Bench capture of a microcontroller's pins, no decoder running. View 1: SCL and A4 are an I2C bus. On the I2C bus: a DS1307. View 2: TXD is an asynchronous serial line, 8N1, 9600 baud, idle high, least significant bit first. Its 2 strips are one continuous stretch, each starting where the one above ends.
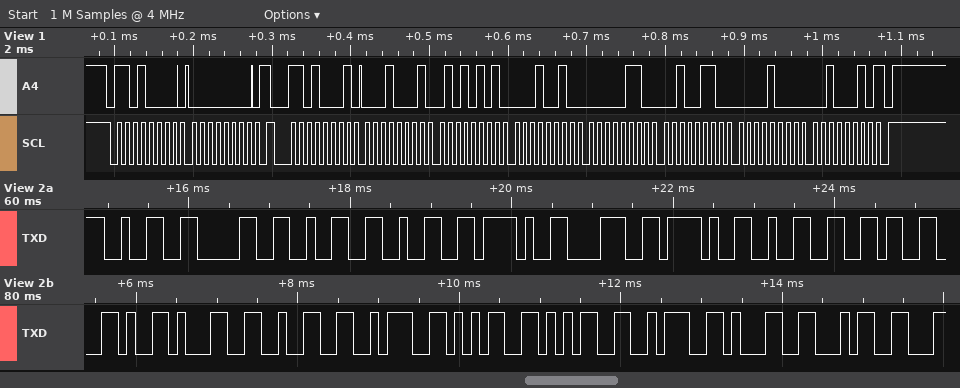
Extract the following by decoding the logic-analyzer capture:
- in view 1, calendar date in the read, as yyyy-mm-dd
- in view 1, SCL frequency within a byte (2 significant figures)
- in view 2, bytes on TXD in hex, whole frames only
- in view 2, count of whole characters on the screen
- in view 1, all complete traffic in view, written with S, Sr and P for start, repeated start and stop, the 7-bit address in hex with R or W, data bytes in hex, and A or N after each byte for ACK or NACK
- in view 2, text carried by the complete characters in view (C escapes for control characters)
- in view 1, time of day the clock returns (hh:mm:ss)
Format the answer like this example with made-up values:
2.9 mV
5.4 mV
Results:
2022-08-26
100 kHz
0x32 0x30 0x32 0x32 0x2F 0x38 0x2F 0x32 0x36 0x2C 0x31 0x32 0x3A 0x35 0x35 0x3A 0x31 0x34
18
S 68W A 00 A Sr 68R A 11 A 55 A 12 A 06 A 26 A 08 A 22 N P
"2022/8/26,12:55:14"
12:55:11
